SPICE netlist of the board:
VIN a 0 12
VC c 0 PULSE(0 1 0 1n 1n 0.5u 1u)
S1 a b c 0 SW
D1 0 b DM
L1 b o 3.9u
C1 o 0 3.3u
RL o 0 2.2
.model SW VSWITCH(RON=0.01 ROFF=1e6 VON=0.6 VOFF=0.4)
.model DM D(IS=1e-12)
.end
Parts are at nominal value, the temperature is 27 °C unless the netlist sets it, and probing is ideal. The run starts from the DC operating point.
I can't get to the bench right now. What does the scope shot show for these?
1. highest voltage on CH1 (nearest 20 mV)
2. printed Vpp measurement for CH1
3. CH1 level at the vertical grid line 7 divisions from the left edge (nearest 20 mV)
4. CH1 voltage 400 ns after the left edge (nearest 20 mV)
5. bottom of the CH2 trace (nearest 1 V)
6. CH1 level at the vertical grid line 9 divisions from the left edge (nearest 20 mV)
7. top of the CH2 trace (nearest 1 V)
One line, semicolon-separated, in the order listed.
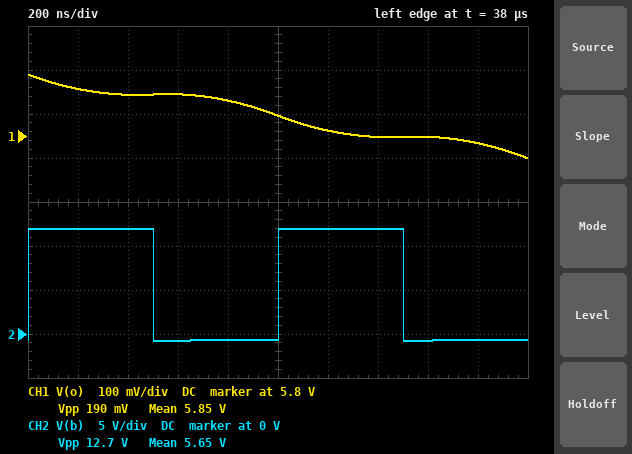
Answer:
5.94 V; 190 mV; 5.80 V; 5.90 V; -1 V; 5.78 V; 12 V
